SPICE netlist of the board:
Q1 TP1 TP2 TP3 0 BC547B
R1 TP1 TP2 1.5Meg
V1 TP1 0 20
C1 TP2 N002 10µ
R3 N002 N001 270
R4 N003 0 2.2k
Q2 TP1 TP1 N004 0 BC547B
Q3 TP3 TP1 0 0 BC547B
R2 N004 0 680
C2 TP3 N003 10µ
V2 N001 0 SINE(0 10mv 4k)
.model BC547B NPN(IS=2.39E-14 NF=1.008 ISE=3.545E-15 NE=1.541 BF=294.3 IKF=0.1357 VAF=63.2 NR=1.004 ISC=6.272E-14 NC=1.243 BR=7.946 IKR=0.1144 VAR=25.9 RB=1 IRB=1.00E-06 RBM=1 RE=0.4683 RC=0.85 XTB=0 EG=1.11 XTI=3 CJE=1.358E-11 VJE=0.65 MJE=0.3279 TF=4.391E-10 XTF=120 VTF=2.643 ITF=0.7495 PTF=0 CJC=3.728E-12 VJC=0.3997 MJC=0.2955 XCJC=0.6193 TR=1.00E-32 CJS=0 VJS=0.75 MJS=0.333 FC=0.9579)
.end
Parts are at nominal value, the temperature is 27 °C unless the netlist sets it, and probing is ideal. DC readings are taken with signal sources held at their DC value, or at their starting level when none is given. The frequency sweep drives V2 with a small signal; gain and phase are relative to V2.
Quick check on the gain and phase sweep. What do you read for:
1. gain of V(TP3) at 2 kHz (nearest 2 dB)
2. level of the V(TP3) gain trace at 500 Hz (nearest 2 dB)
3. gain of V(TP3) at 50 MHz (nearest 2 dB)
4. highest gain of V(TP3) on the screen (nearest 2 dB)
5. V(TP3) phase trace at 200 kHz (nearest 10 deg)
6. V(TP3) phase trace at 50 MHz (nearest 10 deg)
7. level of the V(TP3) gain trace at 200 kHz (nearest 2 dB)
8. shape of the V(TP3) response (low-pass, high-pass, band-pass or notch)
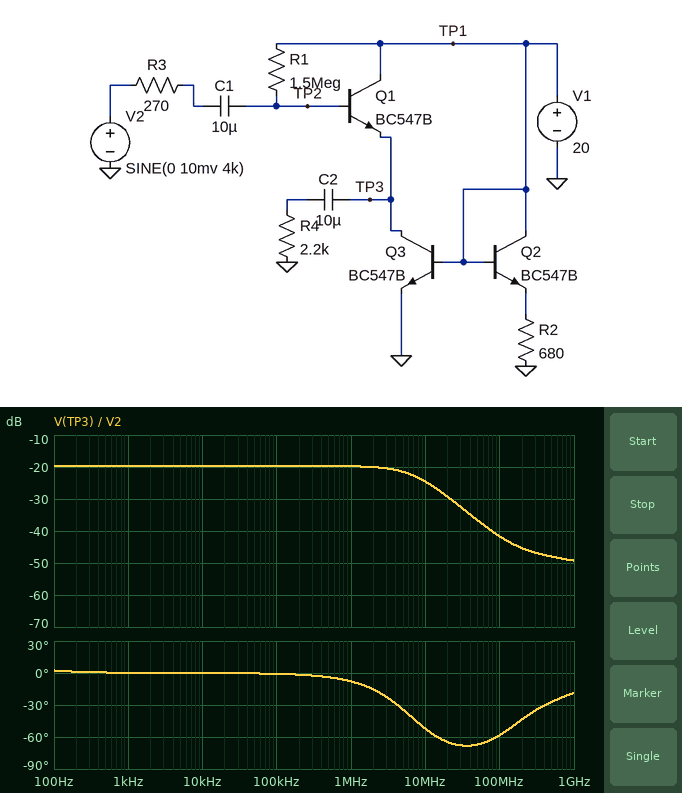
-20 dB
-20 dB
-36 dB
-20 dB
0 deg
-70 deg
-20 dB
low-pass
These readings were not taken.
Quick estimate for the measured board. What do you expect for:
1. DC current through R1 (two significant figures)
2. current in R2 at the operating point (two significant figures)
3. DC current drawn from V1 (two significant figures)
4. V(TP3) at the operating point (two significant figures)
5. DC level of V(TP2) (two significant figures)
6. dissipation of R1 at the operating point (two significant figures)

8.8 µA
28 mA
13 A
6.1 V
6.8 V
120 µW
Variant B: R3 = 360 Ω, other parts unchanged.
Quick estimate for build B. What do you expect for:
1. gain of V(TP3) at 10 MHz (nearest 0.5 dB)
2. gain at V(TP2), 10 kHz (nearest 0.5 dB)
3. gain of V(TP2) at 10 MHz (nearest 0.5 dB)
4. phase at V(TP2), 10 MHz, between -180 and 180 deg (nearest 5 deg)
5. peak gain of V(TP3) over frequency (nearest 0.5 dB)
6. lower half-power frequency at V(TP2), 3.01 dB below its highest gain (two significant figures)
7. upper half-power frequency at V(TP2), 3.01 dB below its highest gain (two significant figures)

-26.5 dB
-1.0 dB
-7.5 dB
-60 deg
-20.0 dB
4.1 Hz
5.3 MHz
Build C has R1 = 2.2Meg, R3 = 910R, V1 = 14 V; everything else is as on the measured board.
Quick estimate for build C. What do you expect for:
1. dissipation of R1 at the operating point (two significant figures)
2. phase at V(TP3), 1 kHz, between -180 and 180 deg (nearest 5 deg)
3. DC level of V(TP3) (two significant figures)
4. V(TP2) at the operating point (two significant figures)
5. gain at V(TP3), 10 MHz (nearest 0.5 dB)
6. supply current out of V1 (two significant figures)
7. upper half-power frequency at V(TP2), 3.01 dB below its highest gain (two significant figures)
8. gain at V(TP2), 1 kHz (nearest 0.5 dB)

38 µW
0 deg
4.2 V
4.9 V
-37.0 dB
8.9 A
3.0 MHz
-1.0 dB
